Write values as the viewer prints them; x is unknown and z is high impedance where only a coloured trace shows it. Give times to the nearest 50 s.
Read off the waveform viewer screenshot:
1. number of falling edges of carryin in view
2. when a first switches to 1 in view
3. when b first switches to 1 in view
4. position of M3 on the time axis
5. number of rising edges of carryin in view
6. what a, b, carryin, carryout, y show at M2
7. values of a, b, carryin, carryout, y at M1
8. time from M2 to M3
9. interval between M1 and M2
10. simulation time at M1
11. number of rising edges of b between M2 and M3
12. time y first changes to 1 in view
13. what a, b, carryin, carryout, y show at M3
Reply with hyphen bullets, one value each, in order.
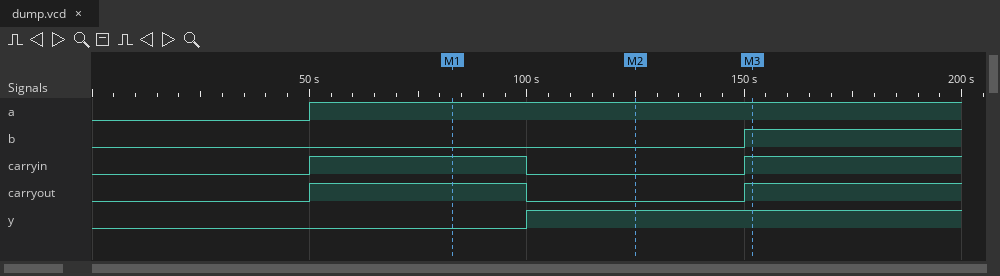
- 1
- 50 s
- 150 s
- 150 s
- 2
- a=1, b=0, carryin=0, carryout=0, y=1
- a=1, b=0, carryin=1, carryout=1, y=0
- 50 s
- 50 s
- 100 s
- 1
- 100 s
- a=1, b=1, carryin=1, carryout=1, y=1
